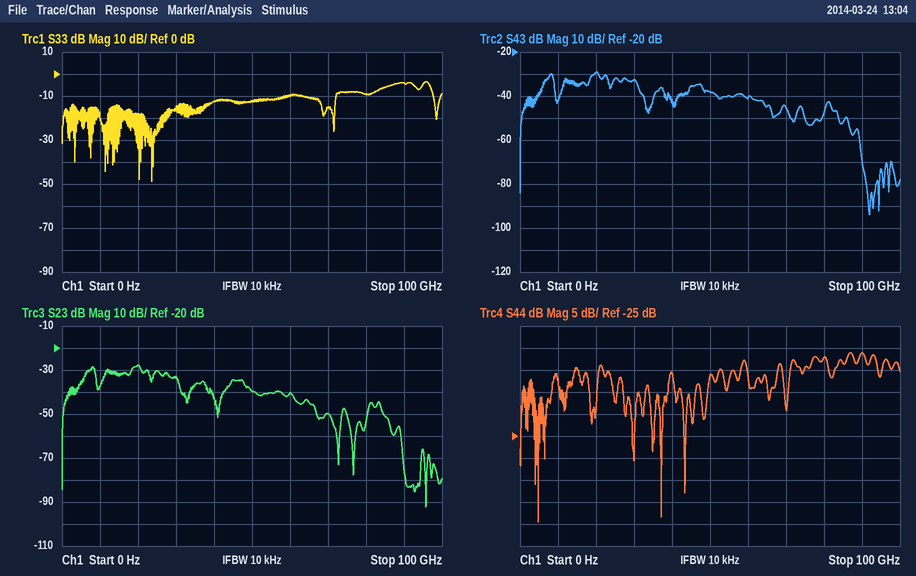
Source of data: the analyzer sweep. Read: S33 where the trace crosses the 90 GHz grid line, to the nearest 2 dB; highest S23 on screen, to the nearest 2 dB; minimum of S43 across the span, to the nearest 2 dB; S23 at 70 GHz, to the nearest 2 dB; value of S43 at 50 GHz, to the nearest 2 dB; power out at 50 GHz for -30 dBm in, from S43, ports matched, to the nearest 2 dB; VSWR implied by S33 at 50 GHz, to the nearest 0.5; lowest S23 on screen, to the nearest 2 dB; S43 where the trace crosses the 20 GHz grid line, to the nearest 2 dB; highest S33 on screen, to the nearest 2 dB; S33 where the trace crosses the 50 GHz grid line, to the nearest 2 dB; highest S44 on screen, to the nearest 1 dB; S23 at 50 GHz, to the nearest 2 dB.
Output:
-4 dB
-28 dB
-94 dB
-50 dB
-38 dB
-68 dBm
1.5
-92 dB
-30 dB
-4 dB
-12 dB
-6 dB
-40 dB
